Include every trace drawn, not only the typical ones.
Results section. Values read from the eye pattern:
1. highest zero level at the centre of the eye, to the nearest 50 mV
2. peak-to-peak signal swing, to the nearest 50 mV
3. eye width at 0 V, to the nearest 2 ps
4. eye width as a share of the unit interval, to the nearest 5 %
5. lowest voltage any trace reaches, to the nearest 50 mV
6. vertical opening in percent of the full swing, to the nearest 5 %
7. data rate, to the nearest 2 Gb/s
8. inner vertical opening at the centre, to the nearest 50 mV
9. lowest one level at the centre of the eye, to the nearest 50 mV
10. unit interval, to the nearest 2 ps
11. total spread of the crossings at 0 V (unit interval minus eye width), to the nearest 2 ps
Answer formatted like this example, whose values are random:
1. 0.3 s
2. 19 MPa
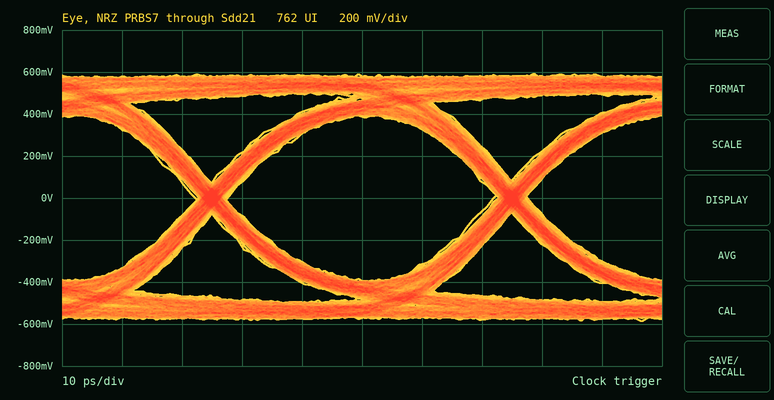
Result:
1. -400 mV
2. 1.20 V
3. 44 ps
4. 90 %
5. -600 mV
6. 65 %
7. 20 Gb/s
8. 800 mV
9. 400 mV
10. 50 ps
11. 6 ps
